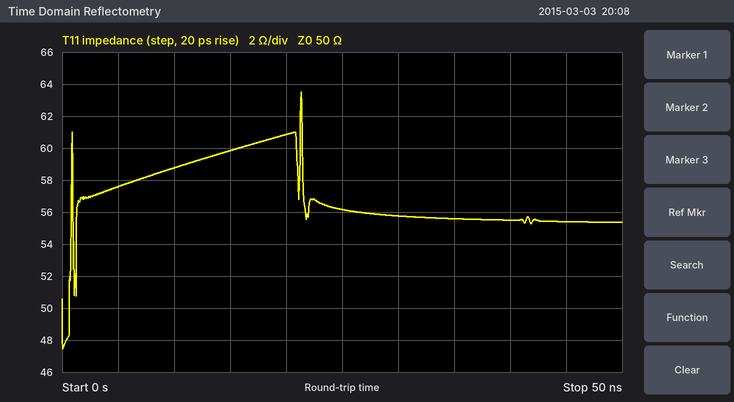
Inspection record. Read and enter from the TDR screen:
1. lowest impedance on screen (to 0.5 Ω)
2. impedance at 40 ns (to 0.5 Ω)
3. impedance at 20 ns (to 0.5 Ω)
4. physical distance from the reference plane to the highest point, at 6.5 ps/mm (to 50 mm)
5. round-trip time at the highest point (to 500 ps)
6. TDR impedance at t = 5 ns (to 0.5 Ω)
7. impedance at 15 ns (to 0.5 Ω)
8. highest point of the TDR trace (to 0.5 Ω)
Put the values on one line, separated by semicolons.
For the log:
47.5 Ω; 55.5 Ω; 61.0 Ω; 1.65 m; 21.5 ns; 57.5 Ω; 60.0 Ω; 63.5 Ω
